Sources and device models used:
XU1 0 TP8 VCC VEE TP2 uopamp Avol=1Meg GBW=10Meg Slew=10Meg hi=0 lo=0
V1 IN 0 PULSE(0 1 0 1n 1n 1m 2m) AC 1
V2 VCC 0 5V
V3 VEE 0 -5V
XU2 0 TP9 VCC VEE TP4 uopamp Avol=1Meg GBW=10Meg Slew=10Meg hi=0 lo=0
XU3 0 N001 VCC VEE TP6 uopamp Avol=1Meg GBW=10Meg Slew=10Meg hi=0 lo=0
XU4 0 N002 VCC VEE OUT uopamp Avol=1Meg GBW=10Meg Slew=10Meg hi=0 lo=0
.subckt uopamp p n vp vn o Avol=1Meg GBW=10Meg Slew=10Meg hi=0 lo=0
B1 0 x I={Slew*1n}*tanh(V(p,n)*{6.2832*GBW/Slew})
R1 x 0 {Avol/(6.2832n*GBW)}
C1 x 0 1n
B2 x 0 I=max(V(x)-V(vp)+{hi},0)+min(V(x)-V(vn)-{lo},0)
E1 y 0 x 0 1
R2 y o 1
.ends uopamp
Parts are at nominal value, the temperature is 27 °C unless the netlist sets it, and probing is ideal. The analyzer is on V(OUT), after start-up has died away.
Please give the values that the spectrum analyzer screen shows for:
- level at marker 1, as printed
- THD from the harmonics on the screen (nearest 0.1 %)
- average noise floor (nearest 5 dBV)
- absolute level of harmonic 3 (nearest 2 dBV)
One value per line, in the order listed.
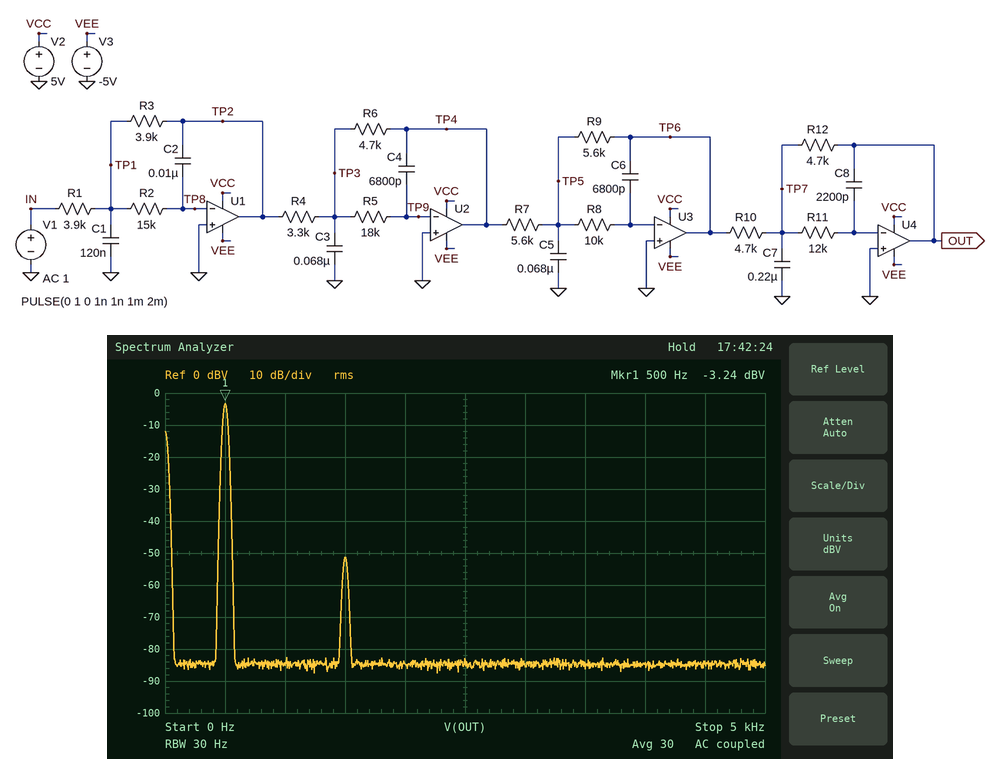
-3.24 dBV
0.4 %
-85 dBV
-52 dBV
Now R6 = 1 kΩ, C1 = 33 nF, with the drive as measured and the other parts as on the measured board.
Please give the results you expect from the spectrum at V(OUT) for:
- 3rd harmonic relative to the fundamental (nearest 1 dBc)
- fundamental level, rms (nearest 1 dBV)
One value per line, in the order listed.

-34 dBc
-17 dBV
